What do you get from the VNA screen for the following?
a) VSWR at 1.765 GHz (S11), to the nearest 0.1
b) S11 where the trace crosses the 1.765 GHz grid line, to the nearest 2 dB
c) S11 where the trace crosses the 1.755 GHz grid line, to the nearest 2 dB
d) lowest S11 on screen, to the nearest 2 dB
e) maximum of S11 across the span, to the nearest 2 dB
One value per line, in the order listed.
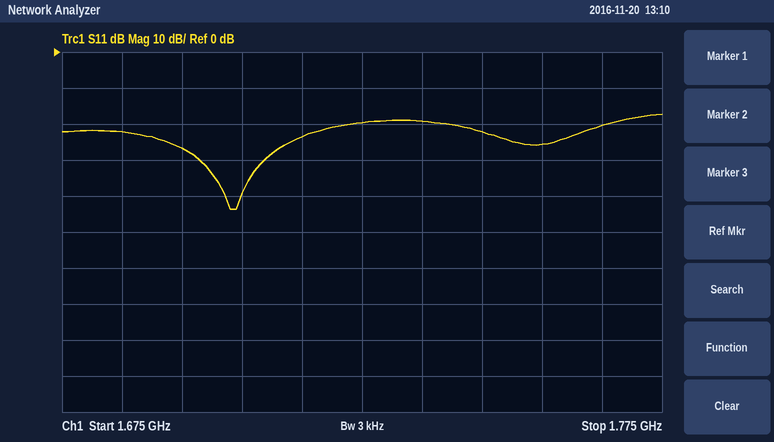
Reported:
1.2
-20 dB
-26 dB
-44 dB
-18 dB
